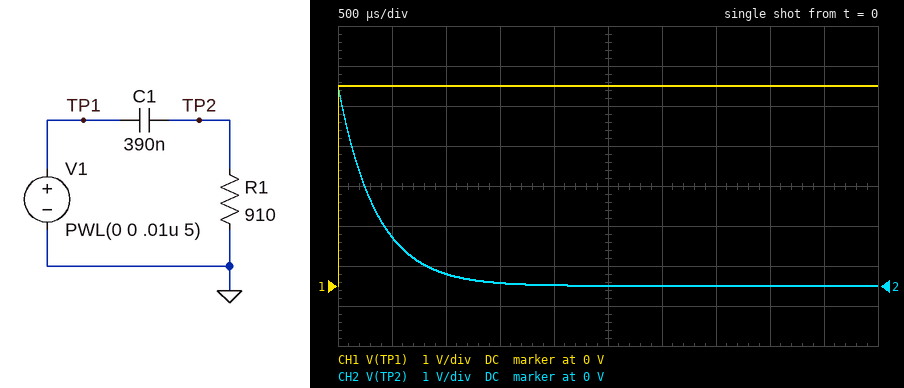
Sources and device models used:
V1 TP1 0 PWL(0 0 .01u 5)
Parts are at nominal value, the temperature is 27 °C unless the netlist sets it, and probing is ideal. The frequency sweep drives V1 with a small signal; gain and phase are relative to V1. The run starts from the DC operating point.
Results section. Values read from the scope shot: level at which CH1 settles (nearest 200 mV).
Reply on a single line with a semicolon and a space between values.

5.0 V
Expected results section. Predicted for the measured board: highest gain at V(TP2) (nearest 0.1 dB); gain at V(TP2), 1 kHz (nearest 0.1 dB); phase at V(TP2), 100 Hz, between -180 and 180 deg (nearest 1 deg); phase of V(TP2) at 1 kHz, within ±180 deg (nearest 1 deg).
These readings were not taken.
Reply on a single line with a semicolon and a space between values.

0 dB; -0.8 dB; 77 deg; 24 deg
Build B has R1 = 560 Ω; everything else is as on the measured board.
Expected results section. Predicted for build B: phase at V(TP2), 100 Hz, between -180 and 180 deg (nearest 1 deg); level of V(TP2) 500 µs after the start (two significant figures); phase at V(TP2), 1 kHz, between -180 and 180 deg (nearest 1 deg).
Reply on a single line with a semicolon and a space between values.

82 deg; 510 mV; 36 deg
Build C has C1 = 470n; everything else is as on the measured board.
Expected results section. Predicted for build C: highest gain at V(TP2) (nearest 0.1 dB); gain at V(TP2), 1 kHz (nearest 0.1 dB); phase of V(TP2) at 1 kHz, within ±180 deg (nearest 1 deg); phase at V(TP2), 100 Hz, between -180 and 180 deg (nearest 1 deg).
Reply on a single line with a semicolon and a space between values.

0 dB; -0.6 dB; 20 deg; 75 deg
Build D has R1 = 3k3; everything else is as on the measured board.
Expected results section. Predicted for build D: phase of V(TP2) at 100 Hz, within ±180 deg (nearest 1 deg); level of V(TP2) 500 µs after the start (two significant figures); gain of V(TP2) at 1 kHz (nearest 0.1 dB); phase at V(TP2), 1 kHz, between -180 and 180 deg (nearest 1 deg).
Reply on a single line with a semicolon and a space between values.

51 deg; 3.4 V; -0.1 dB; 7 deg
